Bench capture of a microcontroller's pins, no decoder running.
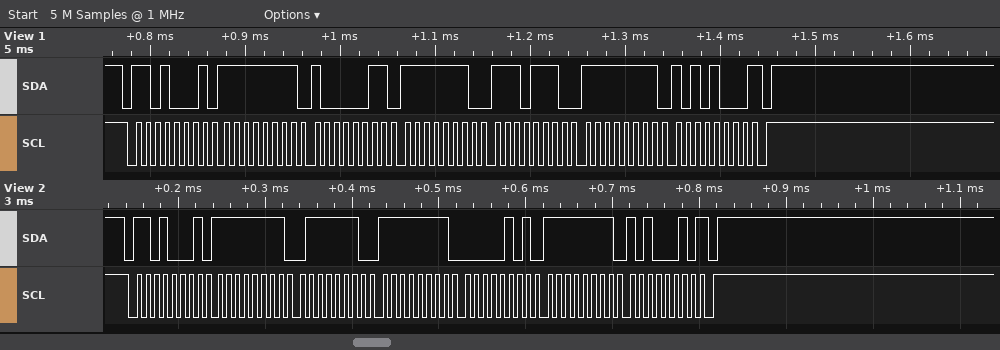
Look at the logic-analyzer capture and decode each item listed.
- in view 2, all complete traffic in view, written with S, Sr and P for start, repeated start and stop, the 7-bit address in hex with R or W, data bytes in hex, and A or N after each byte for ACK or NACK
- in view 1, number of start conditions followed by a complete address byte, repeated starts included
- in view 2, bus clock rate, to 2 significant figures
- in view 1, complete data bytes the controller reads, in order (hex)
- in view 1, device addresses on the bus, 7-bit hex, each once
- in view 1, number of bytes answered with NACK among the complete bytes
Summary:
S 68R A FF A 7E A FF A 05 A FF A A2 N P
1
100 kHz
FF 83 FE EE FF A8
0x68
1
